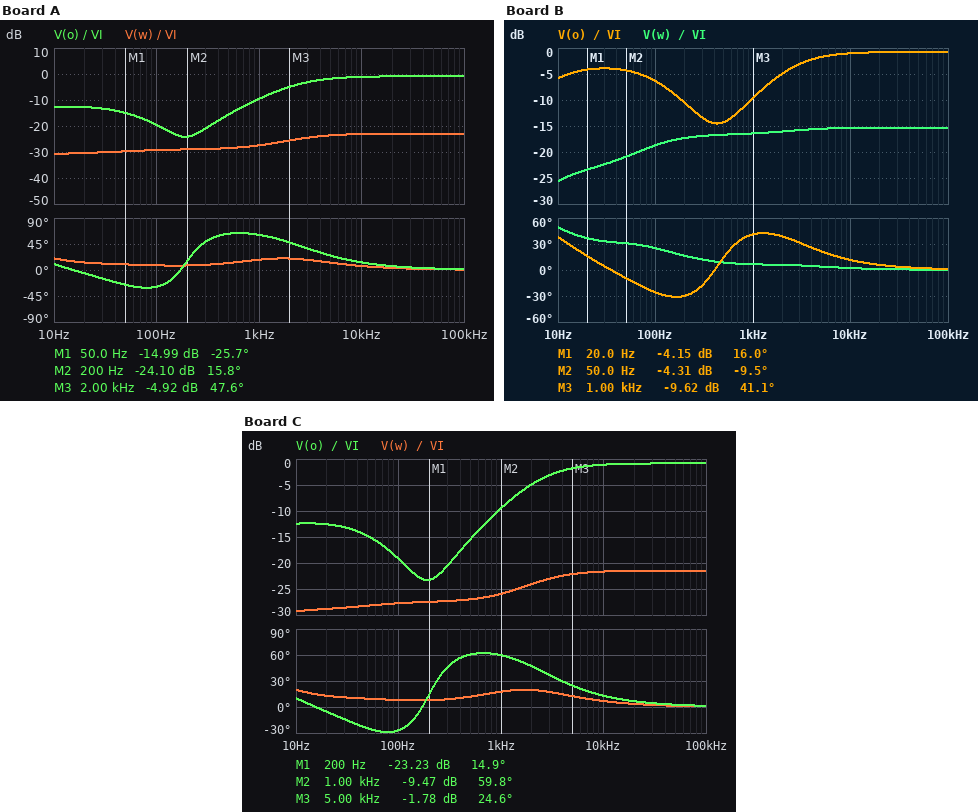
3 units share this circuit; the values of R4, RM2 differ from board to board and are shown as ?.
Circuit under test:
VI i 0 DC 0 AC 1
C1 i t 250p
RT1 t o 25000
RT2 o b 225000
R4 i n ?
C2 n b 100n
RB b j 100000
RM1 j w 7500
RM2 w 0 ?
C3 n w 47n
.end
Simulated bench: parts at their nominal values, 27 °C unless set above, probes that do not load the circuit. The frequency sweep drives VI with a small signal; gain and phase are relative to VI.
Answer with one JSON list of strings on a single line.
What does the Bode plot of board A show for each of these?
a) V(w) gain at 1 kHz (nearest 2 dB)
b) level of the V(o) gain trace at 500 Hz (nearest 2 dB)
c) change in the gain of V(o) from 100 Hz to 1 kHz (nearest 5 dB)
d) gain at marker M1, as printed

["-28 dB", "-16 dB", "10 dB", "-14.99 dB"]
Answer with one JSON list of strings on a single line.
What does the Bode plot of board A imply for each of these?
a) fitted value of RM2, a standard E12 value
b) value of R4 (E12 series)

["10 kΩ", "270 kΩ"]
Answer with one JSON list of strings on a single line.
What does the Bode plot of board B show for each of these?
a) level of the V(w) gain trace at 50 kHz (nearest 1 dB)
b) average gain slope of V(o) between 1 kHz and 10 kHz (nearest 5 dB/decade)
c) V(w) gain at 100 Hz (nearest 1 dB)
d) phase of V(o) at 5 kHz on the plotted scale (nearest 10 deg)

["-15 dB", "10 dB/decade", "-19 dB", "20 deg"]
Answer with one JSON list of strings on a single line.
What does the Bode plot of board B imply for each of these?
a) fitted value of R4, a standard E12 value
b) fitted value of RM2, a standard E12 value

["47 kΩ", "8.2 kΩ"]
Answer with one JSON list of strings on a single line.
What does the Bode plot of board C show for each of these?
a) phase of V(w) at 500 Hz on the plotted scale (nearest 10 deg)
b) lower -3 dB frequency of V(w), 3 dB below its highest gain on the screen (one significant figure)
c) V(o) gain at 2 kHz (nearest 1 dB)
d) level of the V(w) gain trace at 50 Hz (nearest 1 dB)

["10 deg", "2 kHz", "-5 dB", "-28 dB"]
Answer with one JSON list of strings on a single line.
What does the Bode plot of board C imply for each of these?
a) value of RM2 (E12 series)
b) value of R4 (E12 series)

["12 kΩ", "270 kΩ"]
